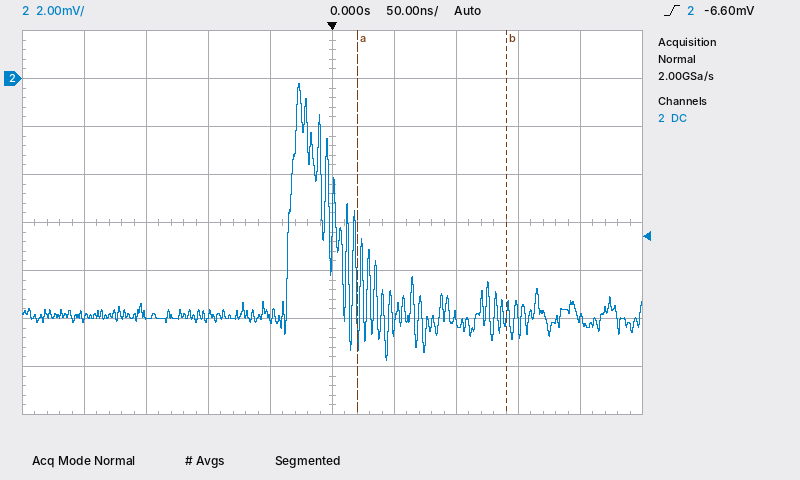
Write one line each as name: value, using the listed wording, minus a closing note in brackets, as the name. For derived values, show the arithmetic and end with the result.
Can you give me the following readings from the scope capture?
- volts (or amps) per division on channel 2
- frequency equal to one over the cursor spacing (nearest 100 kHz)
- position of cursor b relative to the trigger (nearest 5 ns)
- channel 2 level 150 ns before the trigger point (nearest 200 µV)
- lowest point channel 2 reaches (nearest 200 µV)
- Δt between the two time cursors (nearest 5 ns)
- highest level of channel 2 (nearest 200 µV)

volts (or amps) per division on channel 2: 2 mV
frequency equal to one over the cursor spacing: 1 / 120 ns ≈ 8.3 MHz
position of cursor b relative to the trigger: +140 ns
channel 2 level 150 ns before the trigger point: -9.8 mV
lowest point channel 2 reaches: -11.8 mV
Δt between the two time cursors: 120 ns
highest level of channel 2: -200 µV
